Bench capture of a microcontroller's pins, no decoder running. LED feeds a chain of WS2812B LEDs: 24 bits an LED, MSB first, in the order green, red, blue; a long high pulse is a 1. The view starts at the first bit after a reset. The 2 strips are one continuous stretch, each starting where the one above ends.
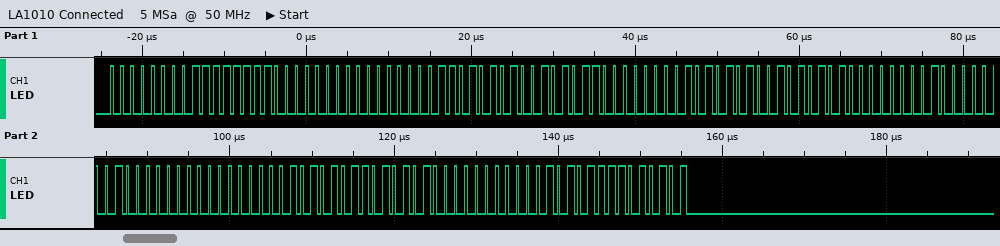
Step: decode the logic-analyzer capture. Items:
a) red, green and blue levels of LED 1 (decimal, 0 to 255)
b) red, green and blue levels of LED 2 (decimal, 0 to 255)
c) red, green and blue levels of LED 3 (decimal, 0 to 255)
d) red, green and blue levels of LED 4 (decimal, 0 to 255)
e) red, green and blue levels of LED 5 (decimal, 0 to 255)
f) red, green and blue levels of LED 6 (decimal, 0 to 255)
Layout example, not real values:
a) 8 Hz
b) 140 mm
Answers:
a) 255, 0, 0
b) 213, 0, 43
c) 170, 0, 85
d) 128, 0, 128
e) 85, 0, 170
f) 43, 0, 213
